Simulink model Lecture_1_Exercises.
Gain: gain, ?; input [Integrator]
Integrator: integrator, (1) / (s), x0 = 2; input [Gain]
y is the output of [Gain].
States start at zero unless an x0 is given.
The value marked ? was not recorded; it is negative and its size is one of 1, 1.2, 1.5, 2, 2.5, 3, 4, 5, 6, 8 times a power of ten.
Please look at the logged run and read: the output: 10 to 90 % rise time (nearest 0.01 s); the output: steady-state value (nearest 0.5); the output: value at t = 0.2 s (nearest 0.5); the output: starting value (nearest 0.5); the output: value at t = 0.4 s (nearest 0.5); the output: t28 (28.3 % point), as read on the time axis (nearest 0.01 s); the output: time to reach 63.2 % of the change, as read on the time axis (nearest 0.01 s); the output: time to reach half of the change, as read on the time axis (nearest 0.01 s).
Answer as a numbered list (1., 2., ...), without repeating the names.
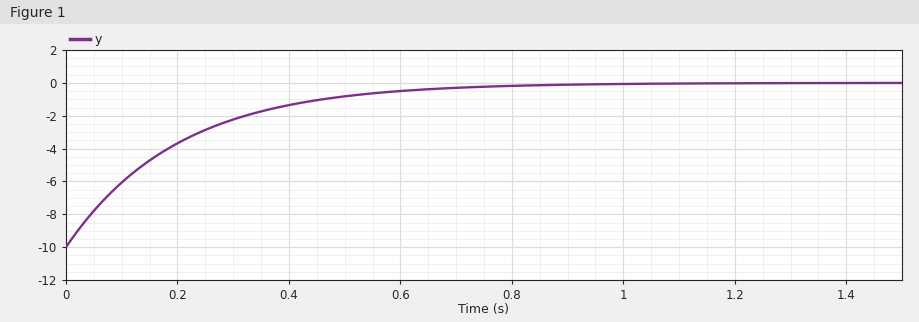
1. 0.44 s
2. 0.0
3. -3.5
4. -10.0
5. -1.5
6. 0.07 s
7. 0.20 s
8. 0.14 s
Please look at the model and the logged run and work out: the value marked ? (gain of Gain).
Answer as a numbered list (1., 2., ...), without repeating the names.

1. -5
